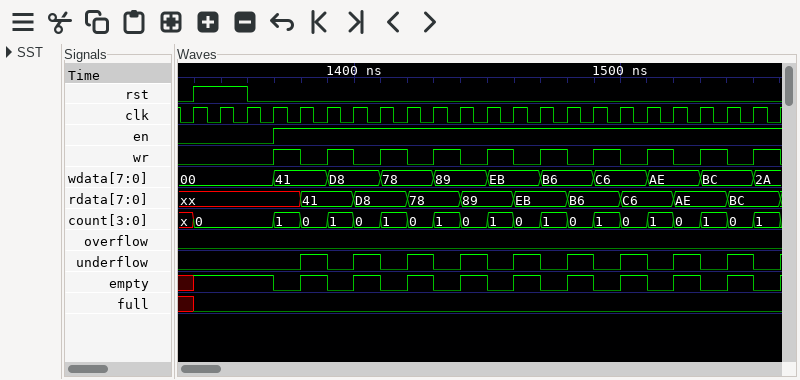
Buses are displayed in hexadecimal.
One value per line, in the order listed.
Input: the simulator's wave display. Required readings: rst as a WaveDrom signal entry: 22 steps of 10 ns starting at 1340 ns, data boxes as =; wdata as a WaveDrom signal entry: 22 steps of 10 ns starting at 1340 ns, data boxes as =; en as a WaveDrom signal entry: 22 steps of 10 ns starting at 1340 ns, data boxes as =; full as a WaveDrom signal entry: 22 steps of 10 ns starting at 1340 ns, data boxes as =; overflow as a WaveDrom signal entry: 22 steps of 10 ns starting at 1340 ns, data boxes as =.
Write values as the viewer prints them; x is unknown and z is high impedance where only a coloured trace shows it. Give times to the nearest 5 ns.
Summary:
{name: 'rst', wave: '1.0...................'}
{name: 'wdata', wave: '=..=.=.=.=.=.=.=.=.=.=', data: '00 41 D8 78 89 EB B6 C6 AE BC 2A'}
{name: 'en', wave: '0..1..................'}
{name: 'full', wave: '0.....................'}
{name: 'overflow', wave: '0.....................'}
